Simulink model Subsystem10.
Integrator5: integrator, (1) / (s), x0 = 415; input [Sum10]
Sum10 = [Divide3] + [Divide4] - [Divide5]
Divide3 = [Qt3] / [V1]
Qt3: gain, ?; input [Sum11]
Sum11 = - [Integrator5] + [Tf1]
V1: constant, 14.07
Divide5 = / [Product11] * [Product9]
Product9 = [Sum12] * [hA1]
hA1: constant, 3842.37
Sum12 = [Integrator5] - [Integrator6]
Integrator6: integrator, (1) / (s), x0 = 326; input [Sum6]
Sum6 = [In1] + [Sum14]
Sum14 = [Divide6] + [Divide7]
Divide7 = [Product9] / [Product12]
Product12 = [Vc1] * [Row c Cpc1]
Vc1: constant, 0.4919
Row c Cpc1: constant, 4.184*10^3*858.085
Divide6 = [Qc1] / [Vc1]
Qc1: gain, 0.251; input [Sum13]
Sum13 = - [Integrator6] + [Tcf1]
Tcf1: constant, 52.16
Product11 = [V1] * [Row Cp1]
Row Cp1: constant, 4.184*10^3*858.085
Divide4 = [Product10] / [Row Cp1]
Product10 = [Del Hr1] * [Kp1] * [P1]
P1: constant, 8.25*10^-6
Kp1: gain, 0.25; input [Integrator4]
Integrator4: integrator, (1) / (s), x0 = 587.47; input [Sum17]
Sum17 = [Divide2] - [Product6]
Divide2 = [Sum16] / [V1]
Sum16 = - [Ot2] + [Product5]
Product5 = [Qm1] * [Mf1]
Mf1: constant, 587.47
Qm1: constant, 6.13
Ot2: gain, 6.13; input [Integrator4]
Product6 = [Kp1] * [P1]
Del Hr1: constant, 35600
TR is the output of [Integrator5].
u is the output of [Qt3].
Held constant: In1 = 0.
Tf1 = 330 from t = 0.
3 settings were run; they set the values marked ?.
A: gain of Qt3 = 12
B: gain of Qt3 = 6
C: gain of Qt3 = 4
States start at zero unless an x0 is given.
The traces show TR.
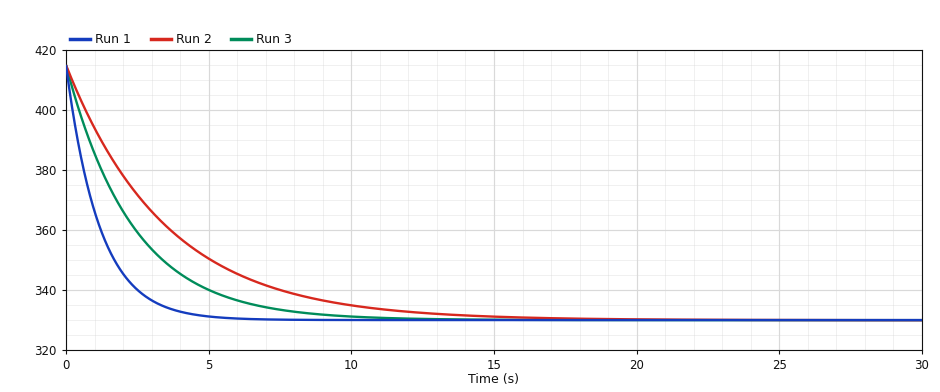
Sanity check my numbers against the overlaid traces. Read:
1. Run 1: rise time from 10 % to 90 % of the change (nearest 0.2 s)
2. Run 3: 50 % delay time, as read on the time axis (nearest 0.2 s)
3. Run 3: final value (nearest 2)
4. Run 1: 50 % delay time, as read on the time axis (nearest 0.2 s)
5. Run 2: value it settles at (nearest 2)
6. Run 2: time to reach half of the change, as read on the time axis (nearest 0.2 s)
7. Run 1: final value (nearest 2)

2.6 s
1.6 s
330
0.8 s
330
2.4 s
330
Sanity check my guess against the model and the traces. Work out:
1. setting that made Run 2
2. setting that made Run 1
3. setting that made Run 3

C
A
B
